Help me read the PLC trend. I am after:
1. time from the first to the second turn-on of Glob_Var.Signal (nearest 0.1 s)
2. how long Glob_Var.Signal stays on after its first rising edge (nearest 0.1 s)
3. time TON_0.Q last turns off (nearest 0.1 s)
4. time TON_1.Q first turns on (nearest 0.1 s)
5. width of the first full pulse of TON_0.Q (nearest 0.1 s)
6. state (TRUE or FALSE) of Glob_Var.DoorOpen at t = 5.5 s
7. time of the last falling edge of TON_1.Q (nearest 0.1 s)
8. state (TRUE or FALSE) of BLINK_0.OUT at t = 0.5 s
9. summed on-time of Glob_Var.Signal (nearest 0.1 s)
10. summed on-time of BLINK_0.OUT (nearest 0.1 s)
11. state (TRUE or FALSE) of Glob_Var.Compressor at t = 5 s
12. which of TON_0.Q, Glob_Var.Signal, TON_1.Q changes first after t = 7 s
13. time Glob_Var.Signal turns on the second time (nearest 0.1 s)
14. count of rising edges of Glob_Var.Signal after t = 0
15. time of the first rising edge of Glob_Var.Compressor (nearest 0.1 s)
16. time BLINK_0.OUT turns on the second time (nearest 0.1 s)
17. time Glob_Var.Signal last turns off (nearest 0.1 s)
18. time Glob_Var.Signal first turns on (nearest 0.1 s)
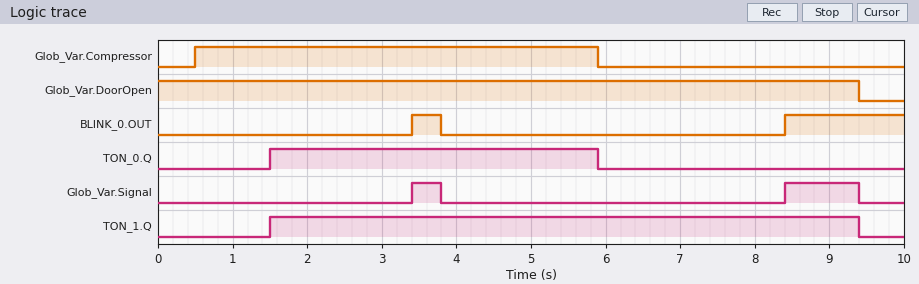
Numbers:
5.0 s
0.4 s
5.9 s
1.5 s
4.4 s
TRUE
9.4 s
FALSE
1.4 s
2.0 s
TRUE
Glob_Var.Signal
8.4 s
2
0.5 s
8.4 s
9.4 s
3.4 s
